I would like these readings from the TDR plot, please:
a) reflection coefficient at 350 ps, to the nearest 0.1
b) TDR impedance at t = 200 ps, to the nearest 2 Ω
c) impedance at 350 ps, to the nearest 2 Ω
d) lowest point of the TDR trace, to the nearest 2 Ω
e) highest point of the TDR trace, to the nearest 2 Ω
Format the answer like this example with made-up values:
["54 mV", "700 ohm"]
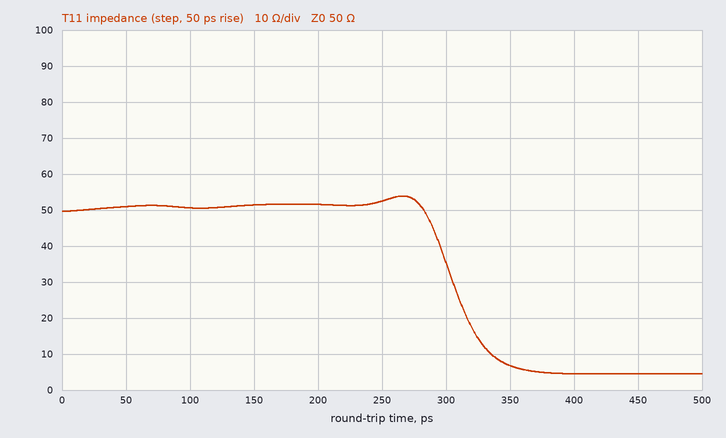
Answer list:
["-0.8", "52 Ω", "6 Ω", "4 Ω", "54 Ω"]
